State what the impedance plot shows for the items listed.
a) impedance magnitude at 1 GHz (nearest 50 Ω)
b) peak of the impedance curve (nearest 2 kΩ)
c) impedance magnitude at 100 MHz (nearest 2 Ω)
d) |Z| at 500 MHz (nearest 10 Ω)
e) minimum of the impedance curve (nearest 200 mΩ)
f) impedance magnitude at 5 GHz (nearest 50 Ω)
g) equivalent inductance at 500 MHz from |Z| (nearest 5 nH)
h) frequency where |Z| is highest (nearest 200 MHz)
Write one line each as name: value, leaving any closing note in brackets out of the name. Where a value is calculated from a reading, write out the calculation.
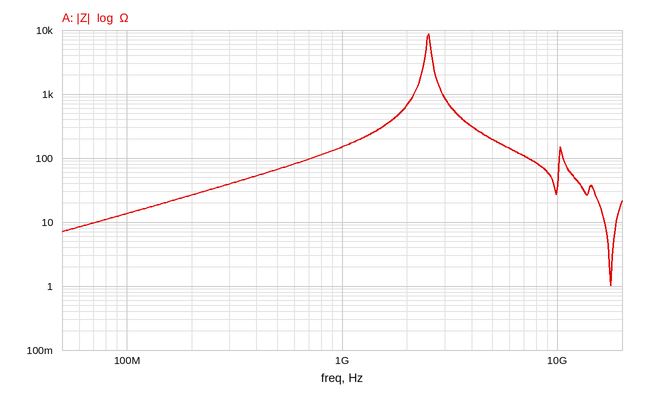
impedance magnitude at 1 GHz: 150 Ω
peak of the impedance curve: 8 kΩ
impedance magnitude at 100 MHz: 14 Ω
|Z| at 500 MHz: 70 Ω
minimum of the impedance curve: 1.0 Ω
impedance magnitude at 5 GHz: 200 Ω
equivalent inductance at 500 MHz from |Z|: L = 70 Ω/(2π × 500 MHz) ≈ 22.3 nH, so 20 nH to the nearest 5 nH
frequency where |Z| is highest: 2.6 GHz
